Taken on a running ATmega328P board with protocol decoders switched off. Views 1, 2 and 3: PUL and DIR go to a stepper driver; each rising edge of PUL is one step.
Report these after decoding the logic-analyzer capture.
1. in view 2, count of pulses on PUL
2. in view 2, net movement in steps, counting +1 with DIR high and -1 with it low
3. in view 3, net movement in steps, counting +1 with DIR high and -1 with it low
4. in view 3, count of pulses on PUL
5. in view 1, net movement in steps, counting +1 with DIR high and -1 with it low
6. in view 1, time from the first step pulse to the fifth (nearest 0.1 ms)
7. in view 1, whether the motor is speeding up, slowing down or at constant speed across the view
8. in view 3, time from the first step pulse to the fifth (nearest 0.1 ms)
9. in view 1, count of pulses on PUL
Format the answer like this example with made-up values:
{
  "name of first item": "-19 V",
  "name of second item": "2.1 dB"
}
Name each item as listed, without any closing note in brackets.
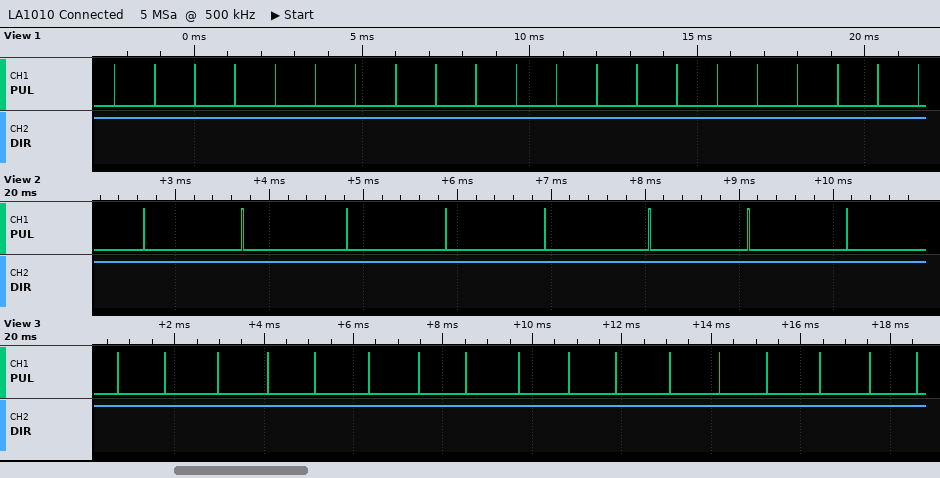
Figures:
{
  "in view 2, count of pulses on PUL": "8",
  "in view 2, net movement in steps, counting +1 with DIR high and -1 with it low": "+8",
  "in view 3, net movement in steps, counting +1 with DIR high and -1 with it low": "+17",
  "in view 3, count of pulses on PUL": "17",
  "in view 1, net movement in steps, counting +1 with DIR high and -1 with it low": "+21",
  "in view 1, time from the first step pulse to the fifth": "4.8 ms",
  "in view 1, whether the motor is speeding up, slowing down or at constant speed across the view": "constant speed",
  "in view 3, time from the first step pulse to the fifth": "4.4 ms",
  "in view 1, count of pulses on PUL": "21"
}
